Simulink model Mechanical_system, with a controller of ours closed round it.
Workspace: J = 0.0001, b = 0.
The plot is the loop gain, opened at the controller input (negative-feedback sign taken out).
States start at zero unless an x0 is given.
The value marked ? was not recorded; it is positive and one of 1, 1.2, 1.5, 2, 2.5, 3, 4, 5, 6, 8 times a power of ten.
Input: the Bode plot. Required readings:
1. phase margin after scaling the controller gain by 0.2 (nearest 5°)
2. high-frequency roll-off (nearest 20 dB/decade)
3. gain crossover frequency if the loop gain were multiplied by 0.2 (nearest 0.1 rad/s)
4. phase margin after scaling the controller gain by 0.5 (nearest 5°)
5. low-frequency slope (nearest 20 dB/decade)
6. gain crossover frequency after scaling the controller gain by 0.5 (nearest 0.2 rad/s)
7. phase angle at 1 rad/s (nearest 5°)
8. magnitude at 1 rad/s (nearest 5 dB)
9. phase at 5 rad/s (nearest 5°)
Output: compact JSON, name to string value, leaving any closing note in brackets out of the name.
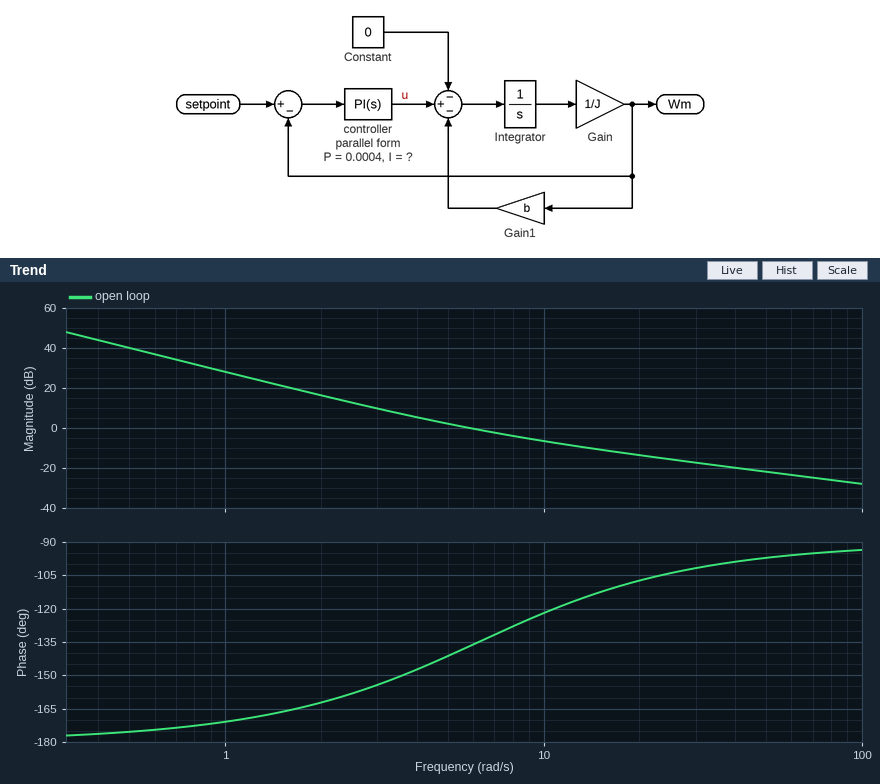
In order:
{"phase margin after scaling the controller gain by 0.2": "20°", "high-frequency roll-off": "-20 dB/decade", "gain crossover frequency if the loop gain were multiplied by 0.2": "2.3 rad/s", "phase margin after scaling the controller gain by 0.5": "30°", "low-frequency slope": "-40 dB/decade", "gain crossover frequency after scaling the controller gain by 0.5": "3.8 rad/s", "phase angle at 1 rad/s": "-170°", "magnitude at 1 rad/s": "30 dB", "phase at 5 rad/s": "-140°"}
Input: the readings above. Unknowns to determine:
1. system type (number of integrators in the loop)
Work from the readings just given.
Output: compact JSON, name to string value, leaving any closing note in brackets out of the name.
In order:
{"system type": "2"}
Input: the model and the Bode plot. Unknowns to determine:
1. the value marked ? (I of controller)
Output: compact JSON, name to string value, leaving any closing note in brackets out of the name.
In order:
{"the value marked ?": "0.0025"}
